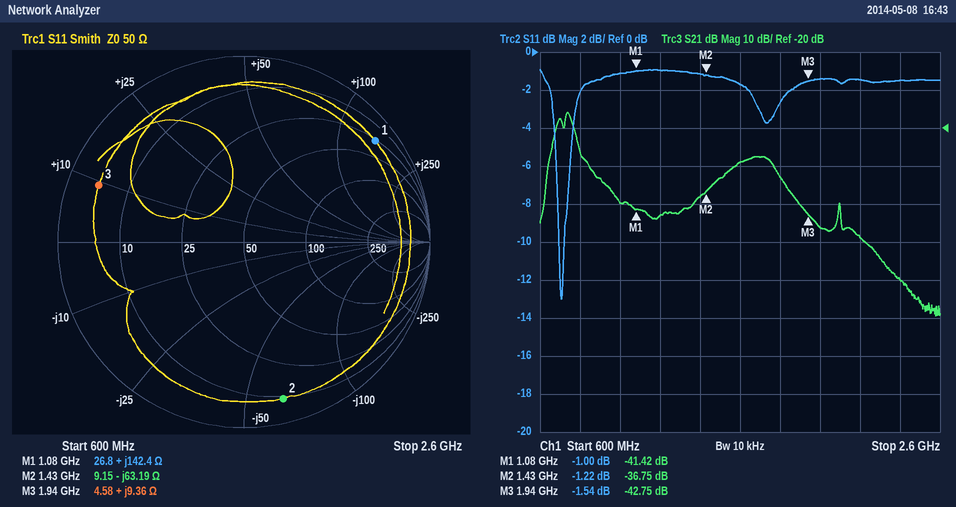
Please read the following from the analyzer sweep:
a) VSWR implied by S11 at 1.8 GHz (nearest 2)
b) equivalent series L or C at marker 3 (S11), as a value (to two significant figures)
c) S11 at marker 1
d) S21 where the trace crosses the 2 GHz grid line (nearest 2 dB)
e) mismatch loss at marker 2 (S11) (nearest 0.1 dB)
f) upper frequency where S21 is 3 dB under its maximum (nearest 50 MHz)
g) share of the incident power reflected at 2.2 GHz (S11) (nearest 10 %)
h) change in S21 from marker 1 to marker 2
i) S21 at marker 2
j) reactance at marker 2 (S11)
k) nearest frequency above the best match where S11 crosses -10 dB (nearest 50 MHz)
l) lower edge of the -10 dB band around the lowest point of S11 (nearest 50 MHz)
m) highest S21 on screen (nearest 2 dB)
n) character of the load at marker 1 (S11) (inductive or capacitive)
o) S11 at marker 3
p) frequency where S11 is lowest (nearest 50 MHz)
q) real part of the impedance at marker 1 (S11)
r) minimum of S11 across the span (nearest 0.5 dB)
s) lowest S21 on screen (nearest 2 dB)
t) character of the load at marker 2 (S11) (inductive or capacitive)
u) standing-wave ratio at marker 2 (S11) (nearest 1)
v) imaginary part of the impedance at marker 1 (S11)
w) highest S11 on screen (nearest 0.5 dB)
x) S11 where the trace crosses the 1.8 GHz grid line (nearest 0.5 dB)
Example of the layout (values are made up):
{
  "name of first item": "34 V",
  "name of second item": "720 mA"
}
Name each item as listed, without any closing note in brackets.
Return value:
{
  "VSWR implied by S11 at 1.8 GHz": "6",
  "equivalent series L or C at marker 3 (S11), as a value": "770 pH",
  "S11 at marker 1": "-1.00 dB",
  "S21 where the trace crosses the 2 GHz grid line": "-46 dB",
  "mismatch loss at marker 2 (S11)": "6.1 dB",
  "upper frequency where S21 is 3 dB under its maximum": "750 MHz",
  "share of the incident power reflected at 2.2 GHz (S11)": "70 %",
  "change in S21 from marker 1 to marker 2": "4.67 dB",
  "S21 at marker 2": "-36.75 dB",
  "reactance at marker 2": "-63.19 Ω",
  "nearest frequency above the best match where S11 crosses -10 dB": "700 MHz",
  "lower edge of the -10 dB band around the lowest point of S11": "700 MHz",
  "highest S21 on screen": "-16 dB",
  "character of the load at marker 1 (S11)": "inductive",
  "S11 at marker 3": "-1.54 dB",
  "frequency where S11 is lowest": "700 MHz",
  "real part of the impedance at marker 1": "26.8 Ω",
  "minimum of S11 across the span": "-13.0 dB",
  "lowest S21 on screen": "-70 dB",
  "character of the load at marker 2 (S11)": "capacitive",
  "standing-wave ratio at marker 2 (S11)": "14",
  "imaginary part of the impedance at marker 1": "+142.4 Ω",
  "highest S11 on screen": "-1.0 dB",
  "S11 where the trace crosses the 1.8 GHz grid line": "-2.5 dB"
}
